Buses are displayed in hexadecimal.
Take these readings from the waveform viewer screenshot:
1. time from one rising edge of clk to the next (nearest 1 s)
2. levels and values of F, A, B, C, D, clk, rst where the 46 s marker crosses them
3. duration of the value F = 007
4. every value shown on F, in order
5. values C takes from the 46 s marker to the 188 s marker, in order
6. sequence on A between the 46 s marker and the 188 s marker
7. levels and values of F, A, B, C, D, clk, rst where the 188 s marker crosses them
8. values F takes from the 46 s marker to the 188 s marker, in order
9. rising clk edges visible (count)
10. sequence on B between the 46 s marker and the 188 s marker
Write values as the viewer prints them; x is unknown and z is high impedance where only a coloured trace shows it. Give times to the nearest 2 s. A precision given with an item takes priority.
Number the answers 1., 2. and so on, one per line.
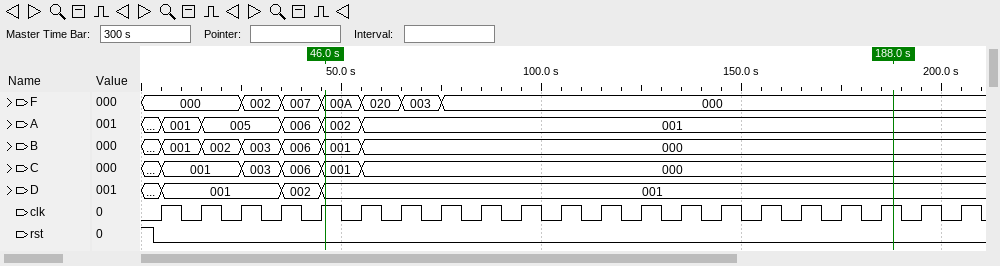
1. 10 s
2. F=00A, A=002, B=001, C=001, D=001, clk=1, rst=0
3. 10 s
4. 000, 002, 007, 00A, 020, 003, 000
5. 001, 000
6. 002, 001
7. F=000, A=001, B=000, C=000, D=001, clk=1, rst=0
8. 00A, 020, 003, 000
9. 21
10. 001, 000
